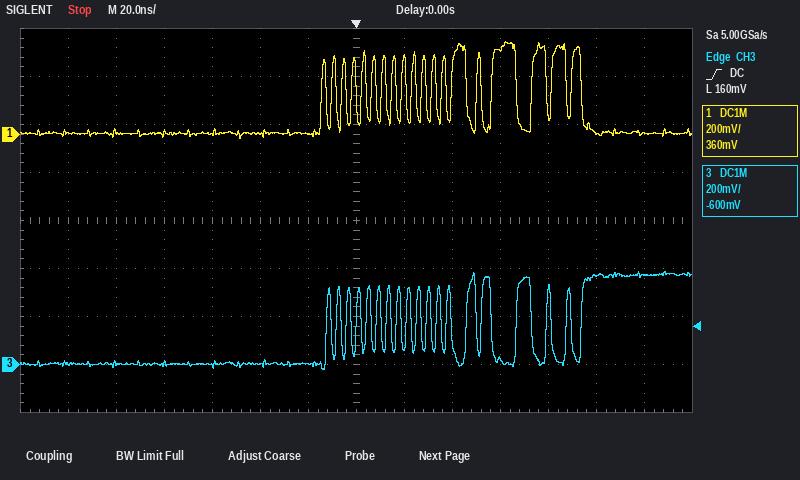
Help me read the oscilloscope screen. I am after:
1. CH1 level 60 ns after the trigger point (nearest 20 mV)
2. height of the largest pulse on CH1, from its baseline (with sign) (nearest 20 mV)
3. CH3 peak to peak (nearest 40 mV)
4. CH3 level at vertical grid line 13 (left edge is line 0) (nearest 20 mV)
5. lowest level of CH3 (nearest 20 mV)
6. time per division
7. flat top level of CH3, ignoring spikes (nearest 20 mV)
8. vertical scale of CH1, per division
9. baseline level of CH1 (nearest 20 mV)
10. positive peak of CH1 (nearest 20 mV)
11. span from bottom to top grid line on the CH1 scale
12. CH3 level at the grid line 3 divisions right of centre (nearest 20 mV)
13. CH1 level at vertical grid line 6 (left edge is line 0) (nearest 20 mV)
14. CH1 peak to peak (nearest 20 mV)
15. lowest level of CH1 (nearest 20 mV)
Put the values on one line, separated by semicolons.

360 mV; +380 mV; 400 mV; 380 mV; -20 mV; 20 ns; 380 mV; 200 mV; 0 mV; 380 mV; 1.6 V; 20 mV; 0 mV; 400 mV; -20 mV
